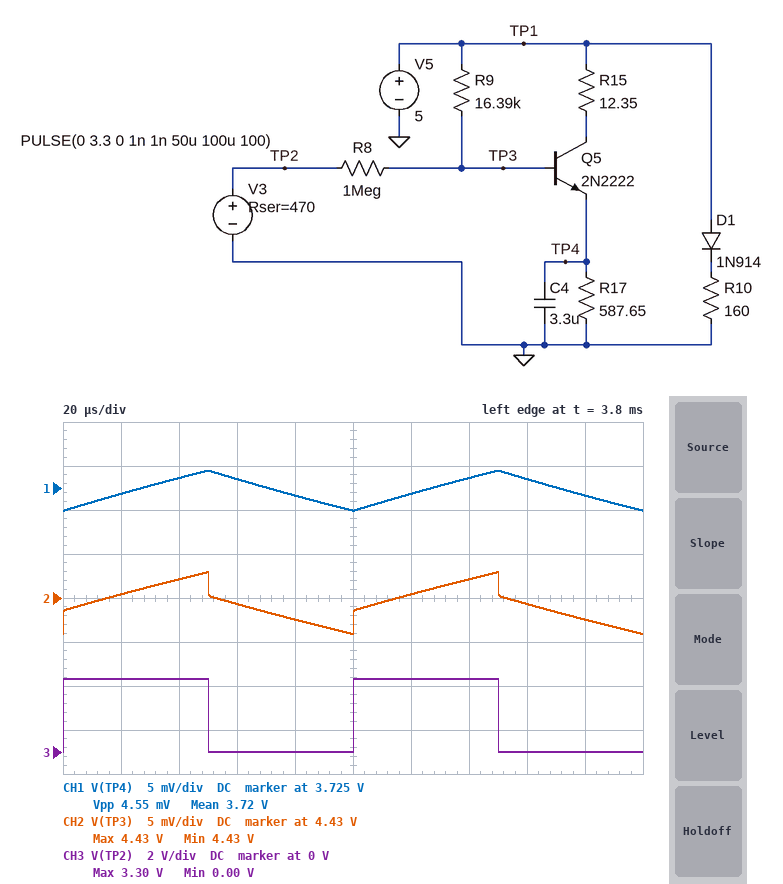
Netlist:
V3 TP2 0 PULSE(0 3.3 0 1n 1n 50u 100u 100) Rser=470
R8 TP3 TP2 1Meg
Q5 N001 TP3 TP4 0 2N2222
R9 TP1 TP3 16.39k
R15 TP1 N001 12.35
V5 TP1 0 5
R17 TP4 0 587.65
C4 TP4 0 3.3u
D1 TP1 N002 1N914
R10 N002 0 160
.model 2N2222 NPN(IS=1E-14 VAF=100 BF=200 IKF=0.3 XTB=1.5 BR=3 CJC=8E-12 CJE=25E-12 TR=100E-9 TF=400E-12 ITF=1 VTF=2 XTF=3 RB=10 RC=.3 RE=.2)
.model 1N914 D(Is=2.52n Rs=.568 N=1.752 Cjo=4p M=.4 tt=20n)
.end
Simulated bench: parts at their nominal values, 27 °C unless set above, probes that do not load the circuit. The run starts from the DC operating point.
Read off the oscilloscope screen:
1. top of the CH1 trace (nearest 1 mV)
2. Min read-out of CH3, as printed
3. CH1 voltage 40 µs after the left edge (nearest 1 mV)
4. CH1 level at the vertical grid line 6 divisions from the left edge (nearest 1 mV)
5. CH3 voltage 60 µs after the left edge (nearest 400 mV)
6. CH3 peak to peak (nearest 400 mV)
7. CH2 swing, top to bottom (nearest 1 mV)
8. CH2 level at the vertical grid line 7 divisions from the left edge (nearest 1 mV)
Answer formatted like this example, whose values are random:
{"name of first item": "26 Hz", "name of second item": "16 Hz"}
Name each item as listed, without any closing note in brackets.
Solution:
{"top of the CH1 trace": "3.727 V", "Min read-out of CH3, as printed": "0.00 V", "CH1 voltage 40 µs after the left edge": "3.726 V", "CH1 level at the vertical grid line 6 divisions from the left edge": "3.724 V", "CH3 voltage 60 µs after the left edge": "0 V", "CH3 peak to peak": "3.2 V", "CH2 swing, top to bottom": "7 mV", "CH2 level at the vertical grid line 7 divisions from the left edge": "4.432 V"}
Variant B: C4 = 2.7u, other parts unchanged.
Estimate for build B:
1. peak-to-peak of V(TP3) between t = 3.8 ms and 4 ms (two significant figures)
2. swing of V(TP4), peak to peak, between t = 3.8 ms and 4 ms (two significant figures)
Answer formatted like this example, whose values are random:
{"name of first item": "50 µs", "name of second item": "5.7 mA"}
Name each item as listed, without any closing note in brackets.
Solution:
{"peak-to-peak of V(TP3) between t = 3.8 ms and 4 ms": "8.0 mV", "swing of V(TP4), peak to peak, between t = 3.8 ms and 4 ms": "5.6 mV"}
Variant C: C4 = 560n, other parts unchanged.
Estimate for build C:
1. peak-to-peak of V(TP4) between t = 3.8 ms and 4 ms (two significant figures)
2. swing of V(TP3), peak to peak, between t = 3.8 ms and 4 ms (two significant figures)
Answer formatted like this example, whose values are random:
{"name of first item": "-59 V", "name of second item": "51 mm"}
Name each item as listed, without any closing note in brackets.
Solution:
{"peak-to-peak of V(TP4) between t = 3.8 ms and 4 ms": "24 mV", "swing of V(TP3), peak to peak, between t = 3.8 ms and 4 ms": "26 mV"}
